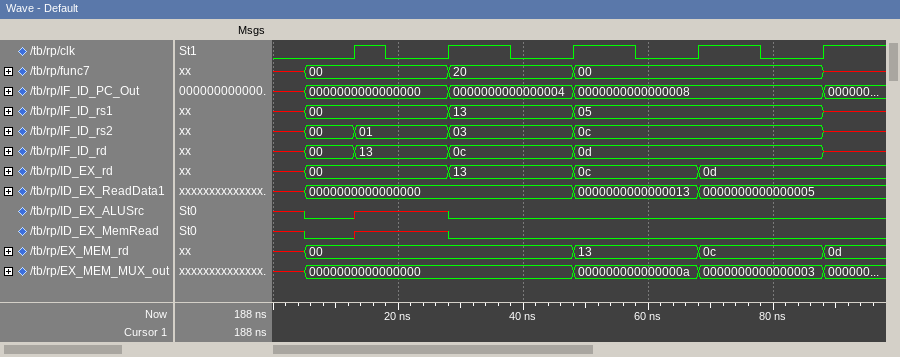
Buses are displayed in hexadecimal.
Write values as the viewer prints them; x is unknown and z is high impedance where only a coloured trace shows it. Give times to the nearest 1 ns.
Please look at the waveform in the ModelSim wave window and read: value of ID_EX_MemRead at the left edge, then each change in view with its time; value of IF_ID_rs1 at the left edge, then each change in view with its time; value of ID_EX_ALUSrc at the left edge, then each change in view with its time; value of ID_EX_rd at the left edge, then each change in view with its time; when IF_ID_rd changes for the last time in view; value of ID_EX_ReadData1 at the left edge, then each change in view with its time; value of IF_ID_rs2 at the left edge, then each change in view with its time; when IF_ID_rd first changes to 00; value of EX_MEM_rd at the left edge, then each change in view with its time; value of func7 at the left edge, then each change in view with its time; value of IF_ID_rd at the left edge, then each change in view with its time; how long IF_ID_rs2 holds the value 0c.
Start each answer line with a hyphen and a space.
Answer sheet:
- x, 0 at 5 ns, x at 13 ns, 0 at 28 ns
- x, 00 at 5 ns, 13 at 28 ns, 05 at 48 ns, x at 88 ns
- x, 0 at 5 ns, x at 13 ns, 0 at 28 ns
- x, 00 at 5 ns, 13 at 28 ns, 0c at 48 ns, 0d at 68 ns
- 88 ns
- x, 0000000000000000 at 5 ns, 0000000000000013 at 48 ns, 0000000000000005 at 68 ns
- x, 00 at 5 ns, 01 at 13 ns, 03 at 28 ns, 0c at 48 ns, x at 88 ns
- 5 ns
- x, 00 at 5 ns, 13 at 48 ns, 0c at 68 ns, 0d at 88 ns
- x, 00 at 5 ns, 20 at 28 ns, 00 at 48 ns, x at 88 ns
- x, 00 at 5 ns, 13 at 13 ns, 0c at 28 ns, 0d at 48 ns, x at 88 ns
- 40 ns
